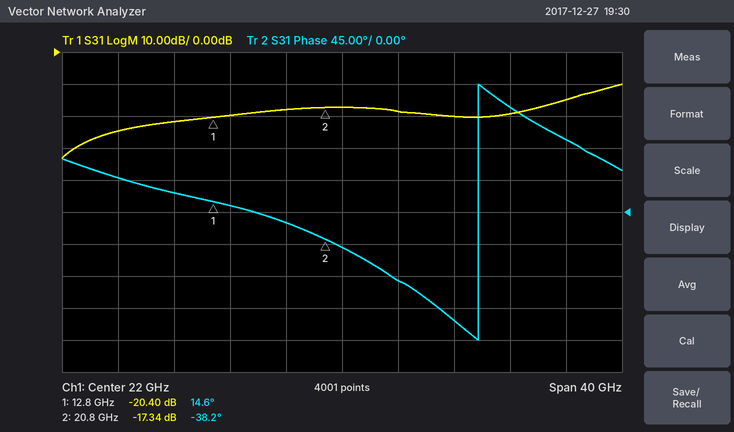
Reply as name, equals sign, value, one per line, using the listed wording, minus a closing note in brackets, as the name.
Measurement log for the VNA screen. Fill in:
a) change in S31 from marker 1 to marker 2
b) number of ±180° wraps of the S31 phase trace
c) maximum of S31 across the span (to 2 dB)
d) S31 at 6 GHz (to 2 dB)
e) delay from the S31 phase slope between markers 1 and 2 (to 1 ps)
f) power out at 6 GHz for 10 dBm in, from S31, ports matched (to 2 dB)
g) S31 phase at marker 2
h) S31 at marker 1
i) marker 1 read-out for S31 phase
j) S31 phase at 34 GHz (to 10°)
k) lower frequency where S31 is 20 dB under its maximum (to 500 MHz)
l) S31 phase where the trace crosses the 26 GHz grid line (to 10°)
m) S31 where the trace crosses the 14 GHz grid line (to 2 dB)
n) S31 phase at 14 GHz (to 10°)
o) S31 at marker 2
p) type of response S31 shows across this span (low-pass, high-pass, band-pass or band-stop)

change in S31 from marker 1 to marker 2 = 3.06 dB
number of ±180° wraps of the S31 phase trace = 1
maximum of S31 across the span = -10 dB
S31 at 6 GHz = -24 dB
delay from the S31 phase slope between markers 1 and 2 = 18 ps
power out at 6 GHz for 10 dBm in, from S31, ports matched = -14 dBm
S31 phase at marker 2 = -38.2°
S31 at marker 1 = -20.40 dB
marker 1 read-out for S31 phase = 14.6°
S31 phase at 34 GHz = 150°
lower frequency where S31 is 20 dB under its maximum = 3.0 GHz
S31 phase where the trace crosses the 26 GHz grid line = -100°
S31 where the trace crosses the 14 GHz grid line = -20 dB
S31 phase at 14 GHz = 10°
S31 at marker 2 = -17.34 dB
type of response S31 shows across this span = high-pass
